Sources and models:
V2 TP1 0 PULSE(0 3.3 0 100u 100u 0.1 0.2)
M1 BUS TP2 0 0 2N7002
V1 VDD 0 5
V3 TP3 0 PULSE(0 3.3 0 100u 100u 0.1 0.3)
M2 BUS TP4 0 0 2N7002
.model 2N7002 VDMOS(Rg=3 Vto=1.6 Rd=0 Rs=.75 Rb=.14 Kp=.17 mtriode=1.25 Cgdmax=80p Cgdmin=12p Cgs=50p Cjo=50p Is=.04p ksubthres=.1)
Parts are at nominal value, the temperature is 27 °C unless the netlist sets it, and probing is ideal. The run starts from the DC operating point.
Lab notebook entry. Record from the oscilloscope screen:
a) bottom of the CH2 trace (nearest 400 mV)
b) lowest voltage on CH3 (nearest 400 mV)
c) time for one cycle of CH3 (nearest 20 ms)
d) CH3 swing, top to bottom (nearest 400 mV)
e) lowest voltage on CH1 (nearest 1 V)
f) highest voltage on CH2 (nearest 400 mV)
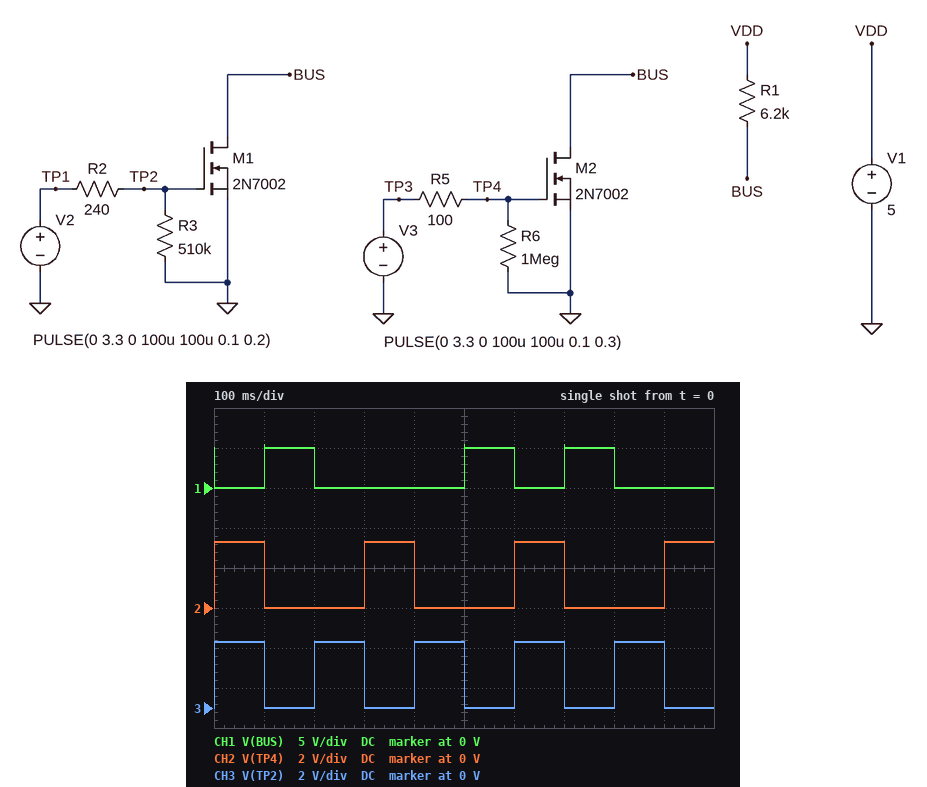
0 V
0 V
200 ms
3.2 V
0 V
3.2 V
